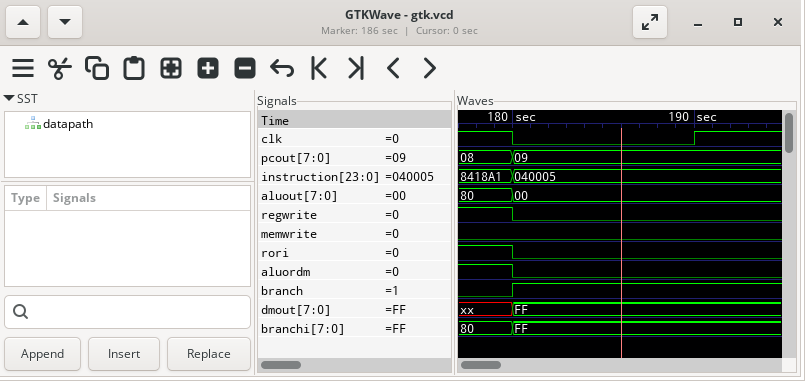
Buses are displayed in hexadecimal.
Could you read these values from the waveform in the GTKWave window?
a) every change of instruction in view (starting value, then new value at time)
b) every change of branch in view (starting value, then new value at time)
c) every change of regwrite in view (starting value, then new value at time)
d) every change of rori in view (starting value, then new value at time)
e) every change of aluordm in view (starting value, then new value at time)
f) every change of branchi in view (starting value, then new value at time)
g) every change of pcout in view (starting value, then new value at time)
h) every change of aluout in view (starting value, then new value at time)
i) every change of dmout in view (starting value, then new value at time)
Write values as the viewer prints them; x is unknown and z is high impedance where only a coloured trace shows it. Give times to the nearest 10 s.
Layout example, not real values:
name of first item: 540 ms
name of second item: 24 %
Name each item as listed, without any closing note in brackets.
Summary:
every change of instruction in view: 8418A1, 040005 at 180 s
every change of branch in view: 0, 1 at 180 s
every change of regwrite in view: 1, 0 at 180 s
every change of rori in view: 1, 0 at 180 s
every change of aluordm in view: 1, 0 at 180 s
every change of branchi in view: 80, FF at 180 s
every change of pcout in view: 08, 09 at 180 s
every change of aluout in view: 80, 00 at 180 s
every change of dmout in view: xx, FF at 180 s
